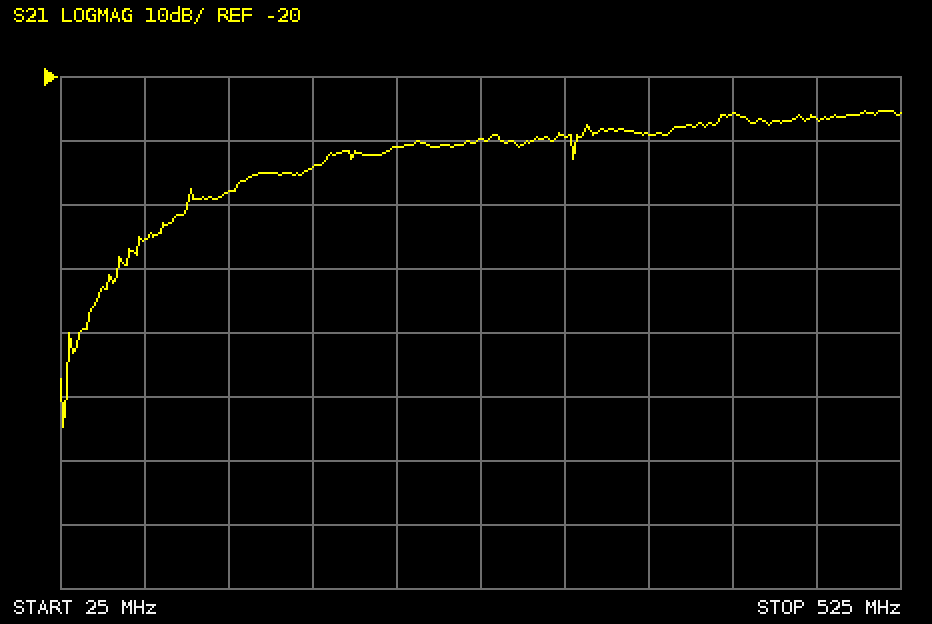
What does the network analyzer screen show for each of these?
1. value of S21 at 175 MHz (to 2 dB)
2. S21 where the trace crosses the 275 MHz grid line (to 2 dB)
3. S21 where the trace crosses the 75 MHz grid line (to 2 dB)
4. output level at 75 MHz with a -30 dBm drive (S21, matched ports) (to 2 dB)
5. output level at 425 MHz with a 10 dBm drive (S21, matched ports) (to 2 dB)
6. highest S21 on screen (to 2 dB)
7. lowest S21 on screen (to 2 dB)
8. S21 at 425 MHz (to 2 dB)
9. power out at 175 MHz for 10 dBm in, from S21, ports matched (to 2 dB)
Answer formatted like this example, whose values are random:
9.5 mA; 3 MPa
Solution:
-34 dB; -30 dB; -46 dB; -76 dBm; -16 dBm; -26 dB; -74 dB; -26 dB; -24 dBm
